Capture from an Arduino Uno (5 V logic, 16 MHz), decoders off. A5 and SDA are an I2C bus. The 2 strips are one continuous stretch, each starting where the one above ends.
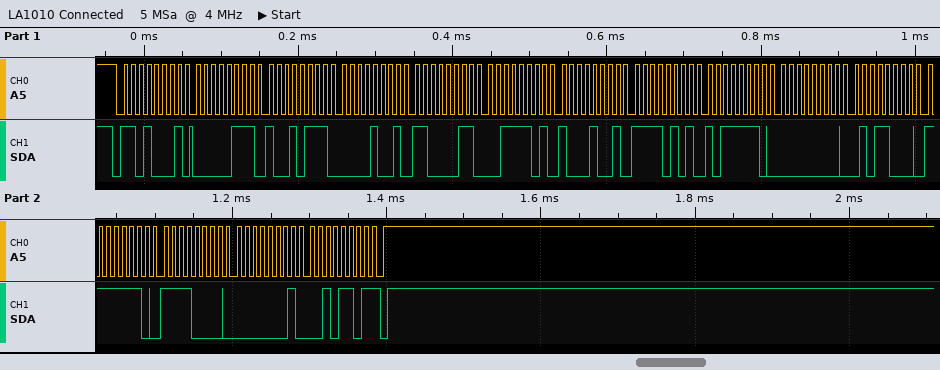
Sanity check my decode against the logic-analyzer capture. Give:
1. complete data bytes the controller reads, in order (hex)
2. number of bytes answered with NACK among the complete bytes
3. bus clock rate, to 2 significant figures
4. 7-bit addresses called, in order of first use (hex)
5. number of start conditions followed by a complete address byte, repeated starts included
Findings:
07 97 09 C3 3D 89 F5 BE 00 58 FE F0 01 2D
1
100 kHz
0x68
1
